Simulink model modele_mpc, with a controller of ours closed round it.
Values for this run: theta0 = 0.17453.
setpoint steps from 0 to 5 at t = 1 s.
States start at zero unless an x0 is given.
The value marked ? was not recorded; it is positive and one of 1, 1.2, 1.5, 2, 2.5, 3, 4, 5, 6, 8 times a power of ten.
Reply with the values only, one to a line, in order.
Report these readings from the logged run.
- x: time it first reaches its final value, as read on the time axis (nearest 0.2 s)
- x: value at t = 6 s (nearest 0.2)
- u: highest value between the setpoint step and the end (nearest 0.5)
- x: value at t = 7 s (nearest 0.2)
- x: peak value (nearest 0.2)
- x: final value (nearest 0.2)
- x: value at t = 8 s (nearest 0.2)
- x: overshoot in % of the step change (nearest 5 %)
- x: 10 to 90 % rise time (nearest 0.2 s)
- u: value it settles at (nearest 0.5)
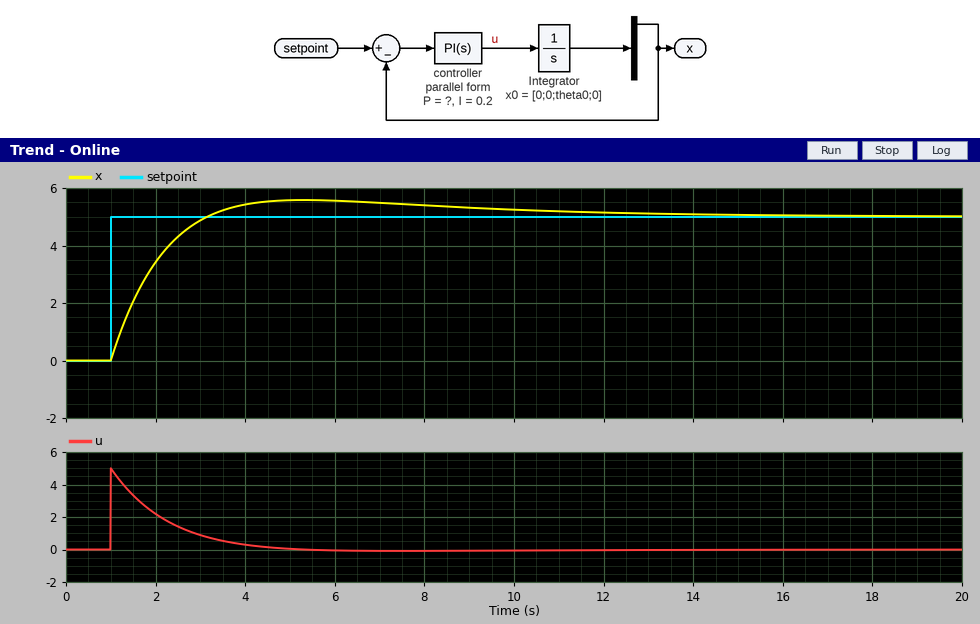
3.2 s
5.6
5.0
5.4
5.6
5.0
5.4
10 %
1.6 s
0.0
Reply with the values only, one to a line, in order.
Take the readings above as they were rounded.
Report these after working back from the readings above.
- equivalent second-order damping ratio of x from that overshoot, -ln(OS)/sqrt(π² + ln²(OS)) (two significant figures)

0.59
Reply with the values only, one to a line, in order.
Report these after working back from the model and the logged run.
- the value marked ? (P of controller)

1
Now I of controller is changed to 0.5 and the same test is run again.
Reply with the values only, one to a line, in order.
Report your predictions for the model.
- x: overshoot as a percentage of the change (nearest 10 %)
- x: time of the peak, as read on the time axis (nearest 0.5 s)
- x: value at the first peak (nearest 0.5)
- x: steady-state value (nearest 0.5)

20 %
4.0 s
6.0
5.0
